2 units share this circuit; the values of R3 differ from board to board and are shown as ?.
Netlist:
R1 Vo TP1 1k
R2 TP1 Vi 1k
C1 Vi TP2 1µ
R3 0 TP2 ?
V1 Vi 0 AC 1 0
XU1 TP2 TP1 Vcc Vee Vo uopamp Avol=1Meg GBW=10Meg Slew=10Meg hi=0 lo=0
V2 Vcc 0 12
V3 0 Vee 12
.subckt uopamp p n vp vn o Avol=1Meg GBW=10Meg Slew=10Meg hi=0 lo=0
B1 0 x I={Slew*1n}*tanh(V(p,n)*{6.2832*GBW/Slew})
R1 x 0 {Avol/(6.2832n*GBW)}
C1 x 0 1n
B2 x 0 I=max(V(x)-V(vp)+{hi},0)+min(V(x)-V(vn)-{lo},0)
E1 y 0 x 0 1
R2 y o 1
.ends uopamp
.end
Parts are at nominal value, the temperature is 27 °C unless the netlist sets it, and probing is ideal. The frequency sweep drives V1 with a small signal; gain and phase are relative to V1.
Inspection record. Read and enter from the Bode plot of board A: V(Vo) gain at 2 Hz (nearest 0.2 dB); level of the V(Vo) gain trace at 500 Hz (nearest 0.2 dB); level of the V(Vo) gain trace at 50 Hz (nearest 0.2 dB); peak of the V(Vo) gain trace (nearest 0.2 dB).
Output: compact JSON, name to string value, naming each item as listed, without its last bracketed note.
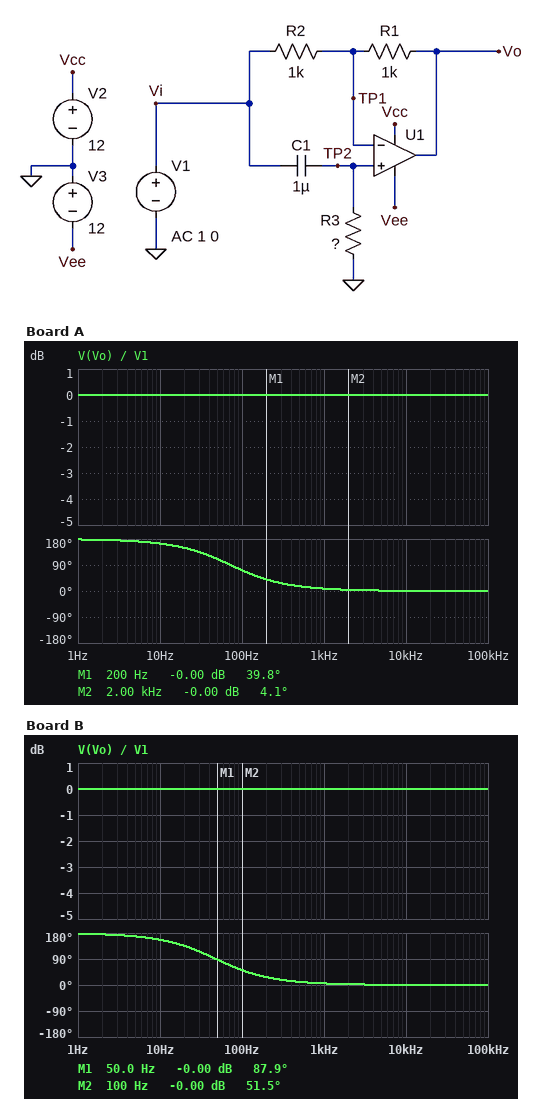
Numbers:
{"V(Vo) gain at 2 Hz": "0 dB", "level of the V(Vo) gain trace at 500 Hz": "0 dB", "level of the V(Vo) gain trace at 50 Hz": "0 dB", "peak of the V(Vo) gain trace": "0 dB"}
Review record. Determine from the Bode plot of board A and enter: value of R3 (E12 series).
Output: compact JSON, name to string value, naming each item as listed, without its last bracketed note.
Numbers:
{"value of R3": "2.2 kΩ"}
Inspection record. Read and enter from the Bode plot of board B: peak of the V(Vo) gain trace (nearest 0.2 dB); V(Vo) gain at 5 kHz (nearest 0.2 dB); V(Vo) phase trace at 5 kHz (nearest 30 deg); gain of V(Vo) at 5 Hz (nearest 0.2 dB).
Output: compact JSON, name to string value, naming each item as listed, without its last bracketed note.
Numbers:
{"peak of the V(Vo) gain trace": "0 dB", "V(Vo) gain at 5 kHz": "0 dB", "V(Vo) phase trace at 5 kHz": "0 deg", "gain of V(Vo) at 5 Hz": "0 dB"}
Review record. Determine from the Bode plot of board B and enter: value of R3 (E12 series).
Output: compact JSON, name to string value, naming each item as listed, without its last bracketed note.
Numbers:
{"value of R3": "3.3 kΩ"}
